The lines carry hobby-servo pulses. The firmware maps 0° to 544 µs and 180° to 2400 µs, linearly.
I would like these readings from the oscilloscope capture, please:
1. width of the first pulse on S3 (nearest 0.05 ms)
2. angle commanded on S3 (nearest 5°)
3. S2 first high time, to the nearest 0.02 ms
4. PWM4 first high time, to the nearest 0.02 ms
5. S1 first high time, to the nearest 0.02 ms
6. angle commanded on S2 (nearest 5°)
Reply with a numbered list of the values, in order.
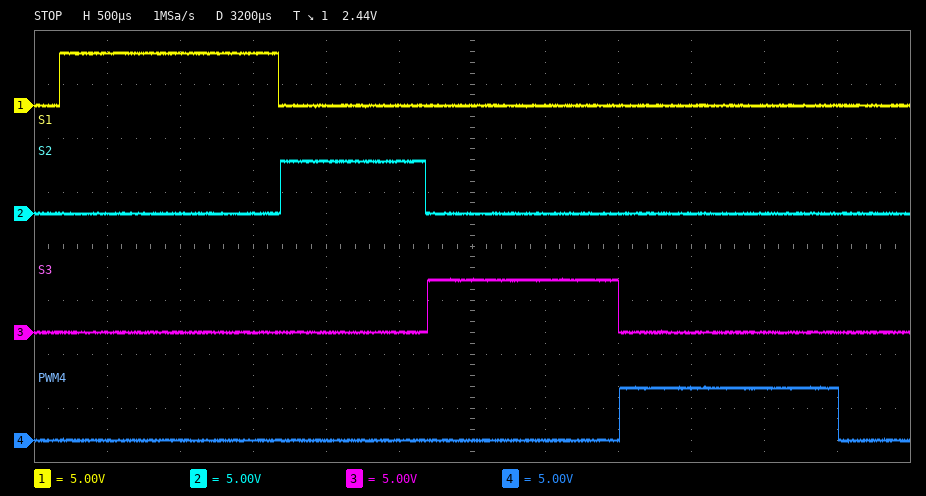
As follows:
1. 1.30 ms
2. 75°
3. 1.00 ms
4. 1.50 ms
5. 1.50 ms
6. 45°
